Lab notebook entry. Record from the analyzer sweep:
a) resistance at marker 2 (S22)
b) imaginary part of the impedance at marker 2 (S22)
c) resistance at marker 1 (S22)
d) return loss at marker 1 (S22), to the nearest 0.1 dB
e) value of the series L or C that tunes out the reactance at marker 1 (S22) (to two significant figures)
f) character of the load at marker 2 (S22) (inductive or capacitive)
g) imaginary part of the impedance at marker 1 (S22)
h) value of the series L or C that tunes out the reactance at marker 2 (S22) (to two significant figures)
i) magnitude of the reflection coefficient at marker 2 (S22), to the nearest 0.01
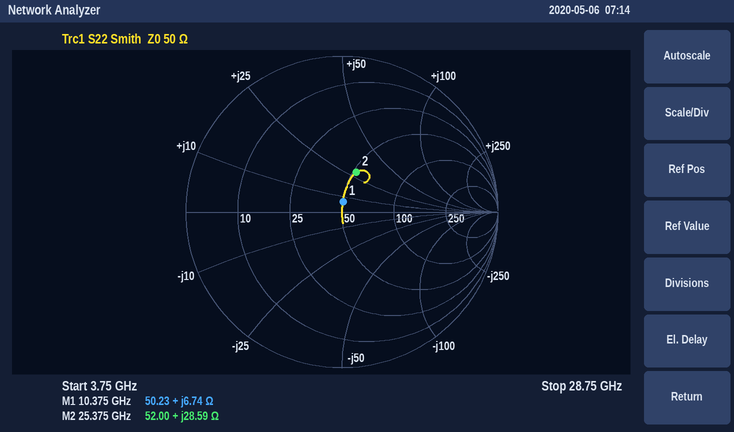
52.00 Ω
+28.59 Ω
50.23 Ω
23.5 dB
2.3 pF
inductive
+6.74 Ω
220 fF
0.27
